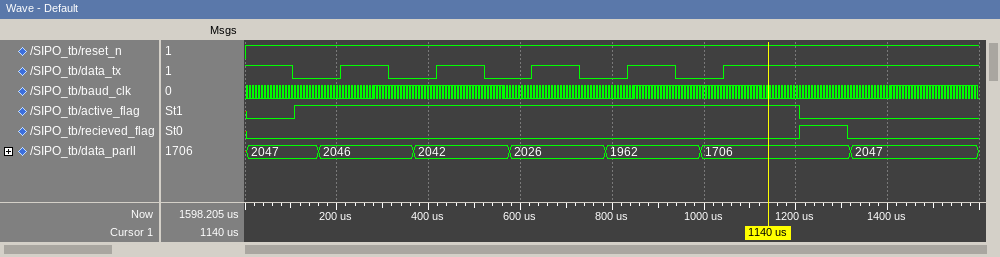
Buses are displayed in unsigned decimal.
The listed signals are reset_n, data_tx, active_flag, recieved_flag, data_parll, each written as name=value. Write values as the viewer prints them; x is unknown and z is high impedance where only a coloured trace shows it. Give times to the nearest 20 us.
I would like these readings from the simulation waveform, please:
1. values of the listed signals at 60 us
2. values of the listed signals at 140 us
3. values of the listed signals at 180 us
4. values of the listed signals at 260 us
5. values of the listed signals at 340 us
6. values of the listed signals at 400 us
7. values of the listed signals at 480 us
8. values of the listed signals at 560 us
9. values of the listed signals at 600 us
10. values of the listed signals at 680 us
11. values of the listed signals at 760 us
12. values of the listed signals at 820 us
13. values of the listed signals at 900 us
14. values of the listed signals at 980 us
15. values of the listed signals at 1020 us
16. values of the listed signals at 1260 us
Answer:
reset_n=1, data_tx=1, active_flag=0, recieved_flag=0, data_parll=2047
reset_n=1, data_tx=0, active_flag=1, recieved_flag=0, data_parll=2047
reset_n=1, data_tx=0, active_flag=1, recieved_flag=0, data_parll=2046
reset_n=1, data_tx=1, active_flag=1, recieved_flag=0, data_parll=2046
reset_n=1, data_tx=0, active_flag=1, recieved_flag=0, data_parll=2046
reset_n=1, data_tx=0, active_flag=1, recieved_flag=0, data_parll=2042
reset_n=1, data_tx=1, active_flag=1, recieved_flag=0, data_parll=2042
reset_n=1, data_tx=0, active_flag=1, recieved_flag=0, data_parll=2042
reset_n=1, data_tx=0, active_flag=1, recieved_flag=0, data_parll=2026
reset_n=1, data_tx=1, active_flag=1, recieved_flag=0, data_parll=2026
reset_n=1, data_tx=0, active_flag=1, recieved_flag=0, data_parll=2026
reset_n=1, data_tx=0, active_flag=1, recieved_flag=0, data_parll=1962
reset_n=1, data_tx=1, active_flag=1, recieved_flag=0, data_parll=1962
reset_n=1, data_tx=0, active_flag=1, recieved_flag=0, data_parll=1962
reset_n=1, data_tx=0, active_flag=1, recieved_flag=0, data_parll=1706
reset_n=1, data_tx=1, active_flag=0, recieved_flag=1, data_parll=1706
